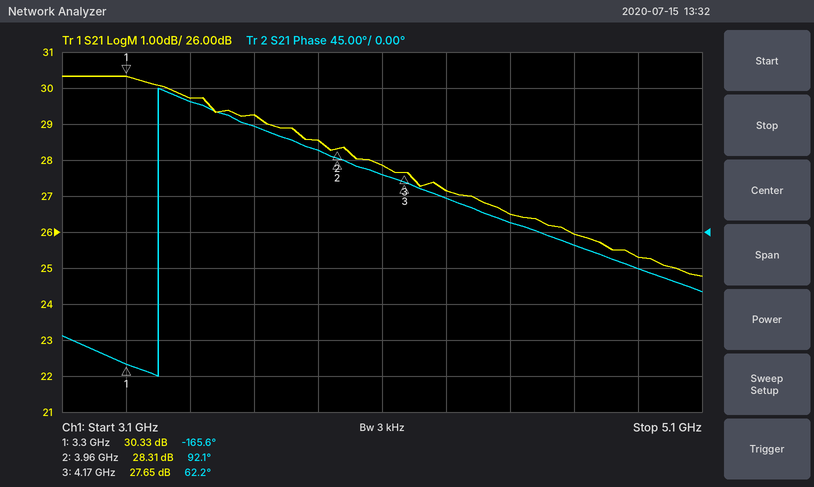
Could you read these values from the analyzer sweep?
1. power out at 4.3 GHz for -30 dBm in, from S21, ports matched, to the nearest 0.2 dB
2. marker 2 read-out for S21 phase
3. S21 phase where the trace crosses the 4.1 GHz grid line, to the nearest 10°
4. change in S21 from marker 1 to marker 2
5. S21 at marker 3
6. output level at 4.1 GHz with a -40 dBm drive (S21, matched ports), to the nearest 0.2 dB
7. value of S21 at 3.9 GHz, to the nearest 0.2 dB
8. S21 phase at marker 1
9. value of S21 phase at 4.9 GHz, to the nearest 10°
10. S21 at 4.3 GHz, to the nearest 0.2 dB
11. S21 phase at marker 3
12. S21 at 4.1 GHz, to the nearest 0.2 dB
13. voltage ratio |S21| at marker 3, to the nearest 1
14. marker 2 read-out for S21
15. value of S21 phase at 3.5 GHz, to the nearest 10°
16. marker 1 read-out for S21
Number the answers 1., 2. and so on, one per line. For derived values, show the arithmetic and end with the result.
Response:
1. -30 dBm + (27.2 dB) = -2.8 dBm
2. 92.1°
3. 70°
4. 28.31 − (30.33) = -2.02 dB
5. 27.65 dB
6. -40 dBm + (27.8 dB) = -12.2 dBm
7. 28.6 dB
8. -165.6°
9. -50°
10. 27.2 dB
11. 62.2°
12. 27.8 dB
13. 10^(27.65/20) ≈ 24
14. 28.31 dB
15. 160°
16. 30.33 dB
